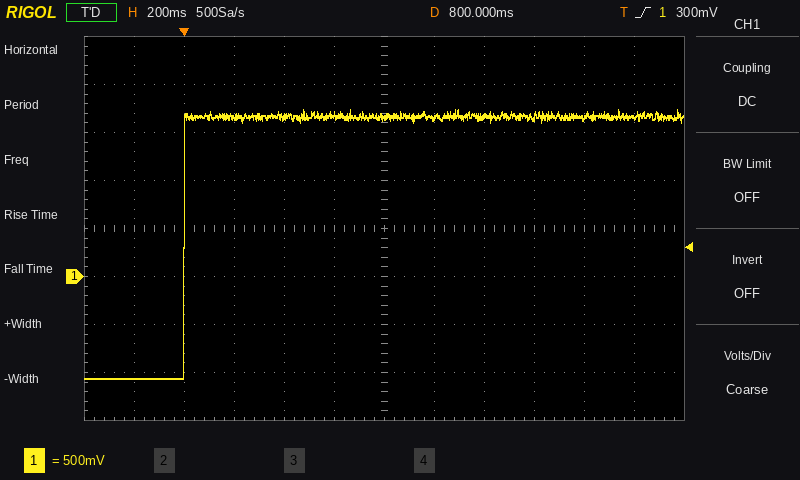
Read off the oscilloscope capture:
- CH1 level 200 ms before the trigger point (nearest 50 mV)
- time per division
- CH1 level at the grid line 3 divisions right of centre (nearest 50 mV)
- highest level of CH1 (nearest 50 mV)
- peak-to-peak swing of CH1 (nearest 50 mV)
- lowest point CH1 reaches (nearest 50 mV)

-1.05 V
200 ms
1.65 V
1.75 V
2.80 V
-1.05 V
